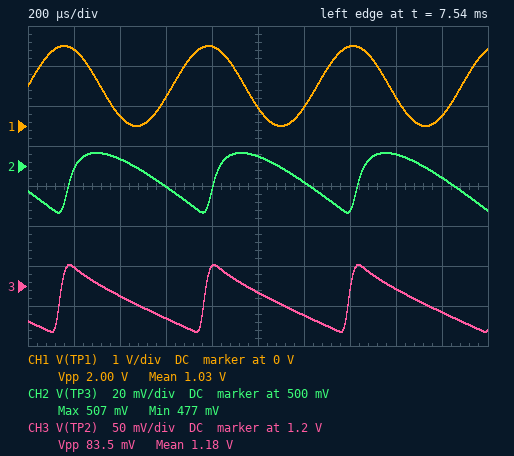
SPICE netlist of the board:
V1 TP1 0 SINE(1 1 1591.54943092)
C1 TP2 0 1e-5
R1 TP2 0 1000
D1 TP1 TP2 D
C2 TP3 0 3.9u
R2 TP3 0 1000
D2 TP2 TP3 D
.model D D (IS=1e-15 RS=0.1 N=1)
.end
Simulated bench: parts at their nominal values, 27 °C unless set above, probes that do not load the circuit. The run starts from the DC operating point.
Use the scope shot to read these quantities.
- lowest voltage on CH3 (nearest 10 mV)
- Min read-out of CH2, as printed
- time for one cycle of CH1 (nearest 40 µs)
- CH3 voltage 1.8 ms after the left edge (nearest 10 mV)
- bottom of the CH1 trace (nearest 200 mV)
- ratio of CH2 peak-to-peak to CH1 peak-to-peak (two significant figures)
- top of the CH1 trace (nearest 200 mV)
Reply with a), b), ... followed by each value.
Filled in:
a) 1.14 V
b) 477 mV
c) 640 µs
d) 1.17 V
e) 0 V
f) 0.015
g) 2.0 V
